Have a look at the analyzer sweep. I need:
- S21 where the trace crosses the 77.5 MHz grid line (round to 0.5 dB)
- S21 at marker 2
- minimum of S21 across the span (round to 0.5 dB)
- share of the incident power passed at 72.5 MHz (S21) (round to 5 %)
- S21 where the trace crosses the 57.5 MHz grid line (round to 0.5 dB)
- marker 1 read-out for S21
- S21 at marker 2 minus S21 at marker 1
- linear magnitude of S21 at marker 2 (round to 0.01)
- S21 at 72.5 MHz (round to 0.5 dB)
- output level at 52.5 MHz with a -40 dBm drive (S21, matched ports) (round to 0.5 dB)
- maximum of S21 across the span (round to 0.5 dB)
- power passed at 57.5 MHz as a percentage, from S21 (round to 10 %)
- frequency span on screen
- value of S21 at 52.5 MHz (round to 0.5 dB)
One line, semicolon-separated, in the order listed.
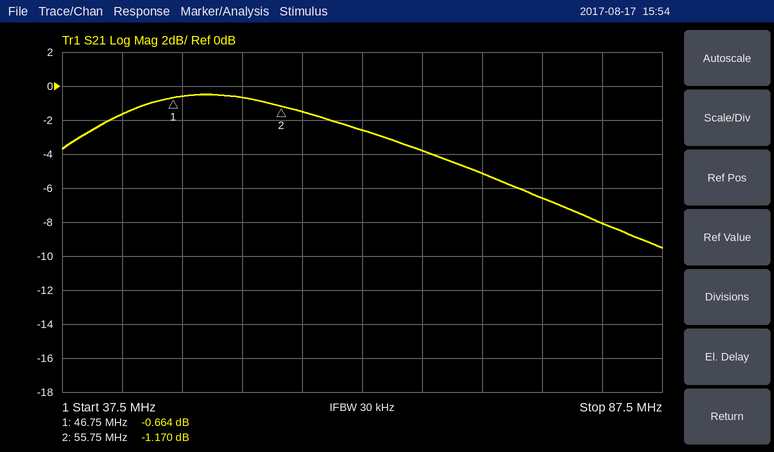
-6.5 dB; -1.170 dB; -9.5 dB; 30 %; -1.5 dB; -0.664 dB; -0.506 dB; 0.87; -5.0 dB; -40.5 dBm; -0.5 dB; 70 %; 50 MHz; -0.5 dB
